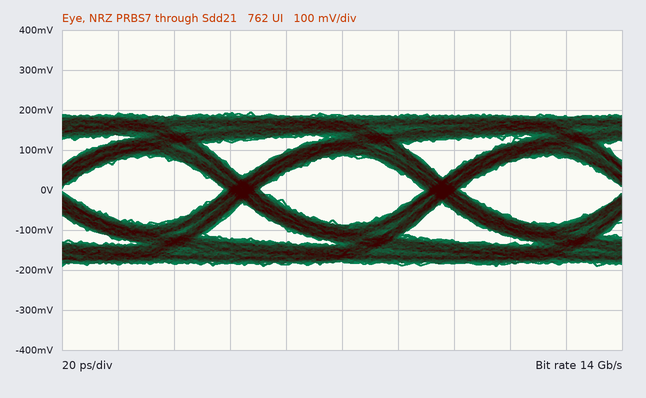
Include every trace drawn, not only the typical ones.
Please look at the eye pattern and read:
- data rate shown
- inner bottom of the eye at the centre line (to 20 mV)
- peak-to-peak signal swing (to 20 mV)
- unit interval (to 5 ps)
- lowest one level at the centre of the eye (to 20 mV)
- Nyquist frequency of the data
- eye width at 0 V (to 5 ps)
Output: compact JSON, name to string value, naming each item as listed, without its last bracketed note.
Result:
{"data rate shown": "14 Gb/s", "inner bottom of the eye at the centre line": "-80 mV", "peak-to-peak signal swing": "380 mV", "unit interval": "70 ps", "lowest one level at the centre of the eye": "80 mV", "Nyquist frequency of the data": "7 GHz", "eye width at 0 V": "60 ps"}
